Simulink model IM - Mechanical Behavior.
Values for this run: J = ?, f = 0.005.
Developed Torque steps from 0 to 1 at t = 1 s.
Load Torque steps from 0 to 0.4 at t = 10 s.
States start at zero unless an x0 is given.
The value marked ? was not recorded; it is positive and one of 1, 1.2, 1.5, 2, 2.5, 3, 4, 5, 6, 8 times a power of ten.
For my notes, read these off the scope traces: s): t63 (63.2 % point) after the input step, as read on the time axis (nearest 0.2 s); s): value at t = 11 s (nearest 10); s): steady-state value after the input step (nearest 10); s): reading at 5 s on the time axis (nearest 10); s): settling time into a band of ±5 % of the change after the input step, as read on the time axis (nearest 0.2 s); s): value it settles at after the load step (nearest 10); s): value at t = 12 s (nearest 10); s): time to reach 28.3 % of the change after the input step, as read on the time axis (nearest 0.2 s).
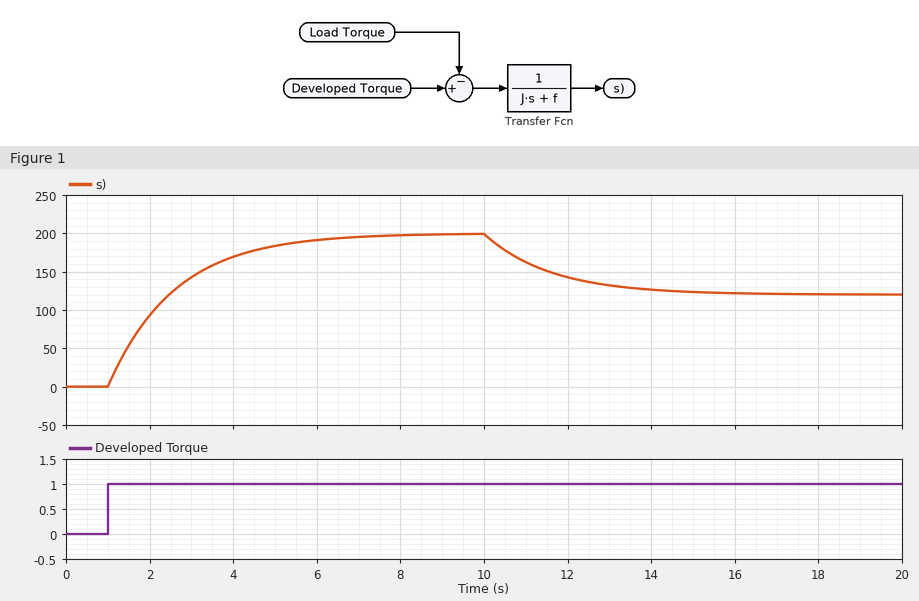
2.6 s
160
200
180
5.8 s
120
140
1.6 s
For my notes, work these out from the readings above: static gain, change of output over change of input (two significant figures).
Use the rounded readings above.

200
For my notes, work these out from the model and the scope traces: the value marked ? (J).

0.008
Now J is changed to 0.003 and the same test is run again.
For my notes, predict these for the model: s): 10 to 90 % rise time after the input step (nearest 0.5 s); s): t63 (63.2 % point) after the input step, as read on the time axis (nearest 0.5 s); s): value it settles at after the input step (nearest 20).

1.5 s
1.5 s
200
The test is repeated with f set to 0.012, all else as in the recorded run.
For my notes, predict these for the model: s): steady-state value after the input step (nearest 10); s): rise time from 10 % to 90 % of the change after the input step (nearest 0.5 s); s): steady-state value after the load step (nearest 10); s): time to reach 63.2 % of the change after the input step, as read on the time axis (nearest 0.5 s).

80
1.5 s
50
1.5 s
